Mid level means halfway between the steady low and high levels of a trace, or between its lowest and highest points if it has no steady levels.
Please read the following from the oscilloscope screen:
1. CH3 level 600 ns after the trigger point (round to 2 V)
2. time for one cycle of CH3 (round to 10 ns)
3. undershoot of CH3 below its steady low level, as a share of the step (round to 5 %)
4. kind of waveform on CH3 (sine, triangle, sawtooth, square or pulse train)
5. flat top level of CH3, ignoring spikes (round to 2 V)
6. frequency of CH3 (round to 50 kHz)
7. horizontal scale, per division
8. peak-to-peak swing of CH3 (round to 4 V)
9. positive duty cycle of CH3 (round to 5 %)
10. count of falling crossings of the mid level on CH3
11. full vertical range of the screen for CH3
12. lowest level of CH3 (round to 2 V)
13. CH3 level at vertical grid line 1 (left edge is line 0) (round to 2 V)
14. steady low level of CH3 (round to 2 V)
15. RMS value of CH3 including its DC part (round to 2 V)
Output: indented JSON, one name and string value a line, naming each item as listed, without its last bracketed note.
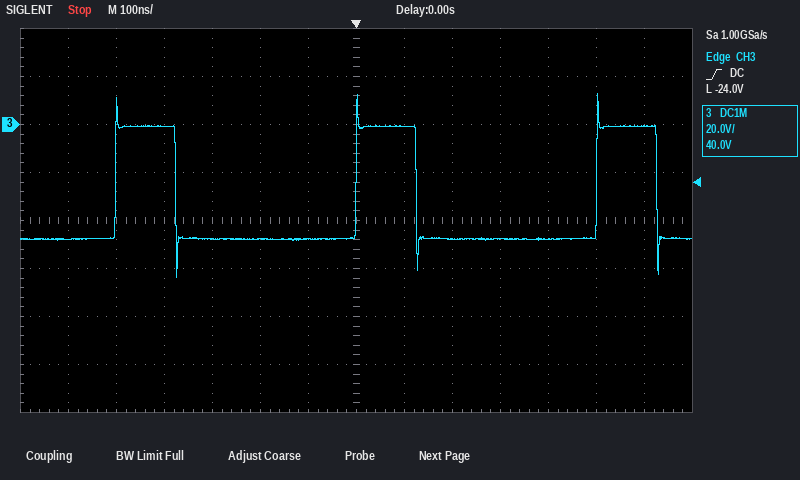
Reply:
{
  "CH3 level 600 ns after the trigger point": "0 V",
  "time for one cycle of CH3": "500 ns",
  "undershoot of CH3 below its steady low level, as a share of the step": "35 %",
  "kind of waveform on CH3": "pulse train",
  "flat top level of CH3, ignoring spikes": "0 V",
  "frequency of CH3": "2.00 MHz",
  "horizontal scale, per division": "100 ns",
  "peak-to-peak swing of CH3": "76 V",
  "positive duty cycle of CH3": "25 %",
  "count of falling crossings of the mid level on CH3": "3",
  "full vertical range of the screen for CH3": "160 V",
  "lowest level of CH3": "-64 V",
  "CH3 level at vertical grid line 1 (left edge is line 0)": "-48 V",
  "steady low level of CH3": "-48 V",
  "RMS value of CH3 including its DC part": "42 V"
}
